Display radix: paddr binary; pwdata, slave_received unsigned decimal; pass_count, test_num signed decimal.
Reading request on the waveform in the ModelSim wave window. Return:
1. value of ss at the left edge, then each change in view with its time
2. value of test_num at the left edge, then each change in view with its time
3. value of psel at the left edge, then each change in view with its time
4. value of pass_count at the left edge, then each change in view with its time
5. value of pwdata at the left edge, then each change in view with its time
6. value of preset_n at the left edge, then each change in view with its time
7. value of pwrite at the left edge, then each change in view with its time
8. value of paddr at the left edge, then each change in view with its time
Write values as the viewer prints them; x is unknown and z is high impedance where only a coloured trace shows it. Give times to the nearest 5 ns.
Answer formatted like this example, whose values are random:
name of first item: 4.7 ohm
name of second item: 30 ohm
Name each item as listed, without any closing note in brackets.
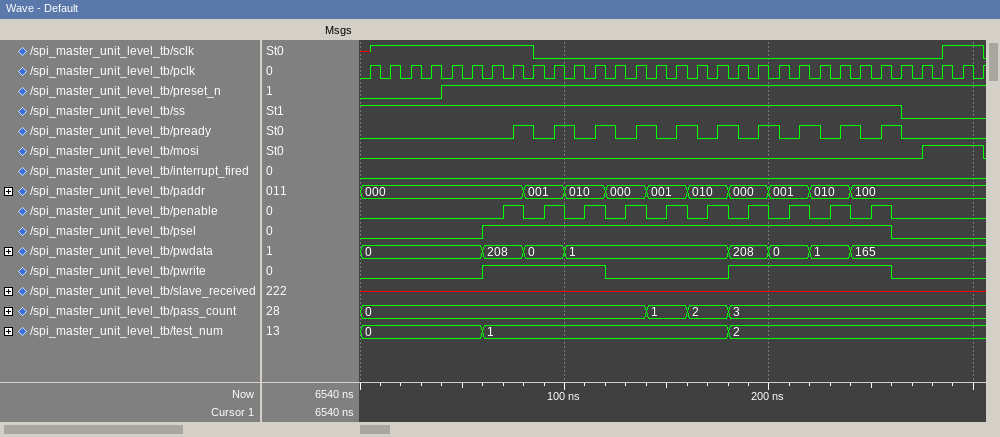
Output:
value of ss at the left edge, then each change in view with its time: 1, 0 at 265 ns
value of test_num at the left edge, then each change in view with its time: 0, 1 at 60 ns, 2 at 180 ns
value of psel at the left edge, then each change in view with its time: 0, 1 at 60 ns, 0 at 260 ns
value of pass_count at the left edge, then each change in view with its time: 0, 1 at 140 ns, 2 at 160 ns, 3 at 180 ns
value of pwdata at the left edge, then each change in view with its time: 0, 208 at 60 ns, 0 at 80 ns, 1 at 100 ns, 208 at 180 ns, 0 at 200 ns, 1 at 220 ns, 165 at 240 ns
value of preset_n at the left edge, then each change in view with its time: 0, 1 at 40 ns
value of pwrite at the left edge, then each change in view with its time: 0, 1 at 60 ns, 0 at 120 ns, 1 at 180 ns, 0 at 260 ns
value of paddr at the left edge, then each change in view with its time: 000, 001 at 80 ns, 010 at 100 ns, 000 at 120 ns, 001 at 140 ns, 010 at 160 ns, 000 at 180 ns, 001 at 200 ns, 010 at 220 ns, 100 at 240 ns
